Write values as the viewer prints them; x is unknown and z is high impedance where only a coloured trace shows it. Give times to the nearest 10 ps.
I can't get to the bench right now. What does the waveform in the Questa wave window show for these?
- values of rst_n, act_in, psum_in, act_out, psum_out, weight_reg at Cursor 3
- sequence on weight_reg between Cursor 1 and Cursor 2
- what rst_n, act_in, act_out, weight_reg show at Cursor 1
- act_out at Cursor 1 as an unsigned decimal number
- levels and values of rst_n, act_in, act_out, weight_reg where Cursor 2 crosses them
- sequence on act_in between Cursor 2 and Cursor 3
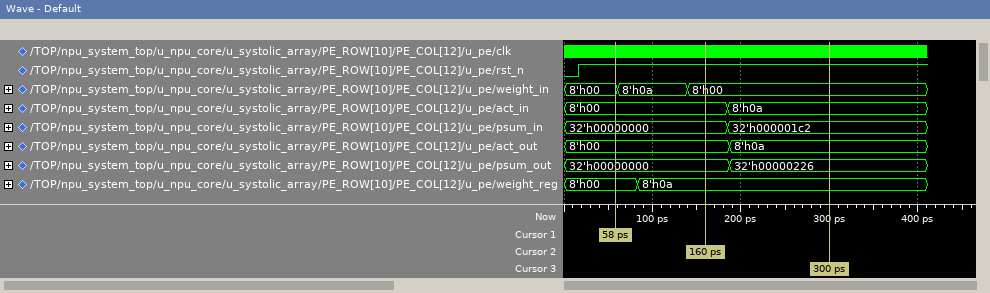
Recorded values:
rst_n=1, act_in=8'h0a, psum_in=32'h000001c2, act_out=8'h0a, psum_out=32'h00000226, weight_reg=8'h0a
8'h00, 8'h0a
rst_n=1, act_in=8'h00, act_out=8'h00, weight_reg=8'h00
0
rst_n=1, act_in=8'h00, act_out=8'h00, weight_reg=8'h0a
8'h00, 8'h0a
